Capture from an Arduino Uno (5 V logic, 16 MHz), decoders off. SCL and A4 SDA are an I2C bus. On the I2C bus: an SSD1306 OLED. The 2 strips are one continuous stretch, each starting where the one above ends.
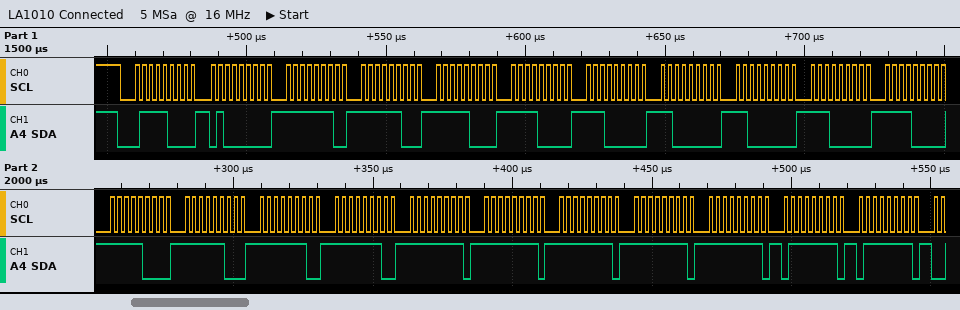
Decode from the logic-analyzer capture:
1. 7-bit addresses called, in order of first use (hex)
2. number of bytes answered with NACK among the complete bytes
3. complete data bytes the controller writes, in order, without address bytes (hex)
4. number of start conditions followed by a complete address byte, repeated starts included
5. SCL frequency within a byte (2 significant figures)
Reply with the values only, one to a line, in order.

0x3C
0
40 FE FC F8 F0 E0 C0 C0 E0 F0 F8 FC FE FE FF FF FF FF FF 7F 7F
1
400 kHz
